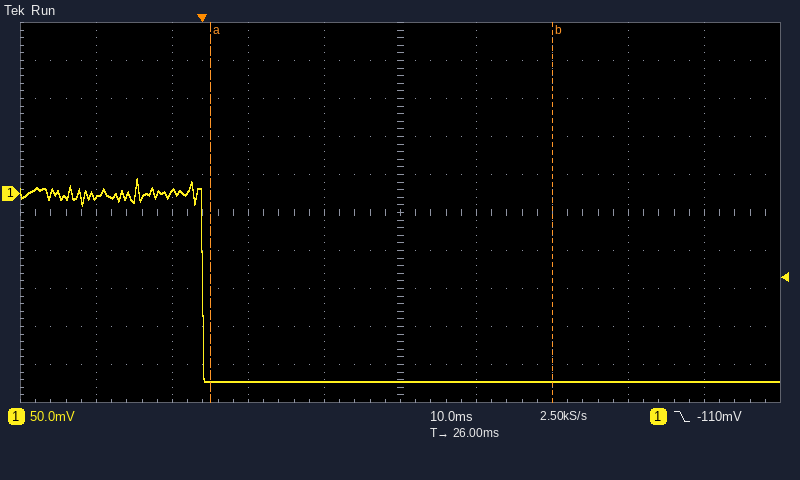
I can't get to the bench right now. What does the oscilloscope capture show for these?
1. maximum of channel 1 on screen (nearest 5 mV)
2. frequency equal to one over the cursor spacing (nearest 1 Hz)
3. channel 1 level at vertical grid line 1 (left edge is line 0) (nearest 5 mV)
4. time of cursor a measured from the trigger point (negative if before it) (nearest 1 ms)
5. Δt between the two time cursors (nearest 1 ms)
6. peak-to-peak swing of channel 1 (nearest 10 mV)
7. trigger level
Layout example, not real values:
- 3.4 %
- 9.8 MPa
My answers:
- 20 mV
- 22 Hz
- -5 mV
- +1 ms
- 45 ms
- 270 mV
- -110 mV
